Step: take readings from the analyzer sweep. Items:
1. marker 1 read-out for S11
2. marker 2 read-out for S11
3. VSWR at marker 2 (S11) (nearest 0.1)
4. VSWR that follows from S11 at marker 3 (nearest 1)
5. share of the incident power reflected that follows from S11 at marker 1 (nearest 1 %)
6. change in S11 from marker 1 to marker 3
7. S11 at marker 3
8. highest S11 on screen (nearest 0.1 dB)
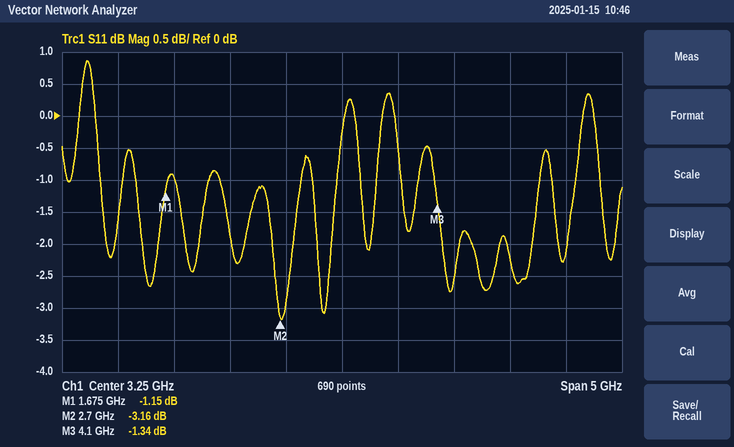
-1.15 dB
-3.16 dB
5.6
13
77 %
-0.19 dB
-1.34 dB
0.9 dB
